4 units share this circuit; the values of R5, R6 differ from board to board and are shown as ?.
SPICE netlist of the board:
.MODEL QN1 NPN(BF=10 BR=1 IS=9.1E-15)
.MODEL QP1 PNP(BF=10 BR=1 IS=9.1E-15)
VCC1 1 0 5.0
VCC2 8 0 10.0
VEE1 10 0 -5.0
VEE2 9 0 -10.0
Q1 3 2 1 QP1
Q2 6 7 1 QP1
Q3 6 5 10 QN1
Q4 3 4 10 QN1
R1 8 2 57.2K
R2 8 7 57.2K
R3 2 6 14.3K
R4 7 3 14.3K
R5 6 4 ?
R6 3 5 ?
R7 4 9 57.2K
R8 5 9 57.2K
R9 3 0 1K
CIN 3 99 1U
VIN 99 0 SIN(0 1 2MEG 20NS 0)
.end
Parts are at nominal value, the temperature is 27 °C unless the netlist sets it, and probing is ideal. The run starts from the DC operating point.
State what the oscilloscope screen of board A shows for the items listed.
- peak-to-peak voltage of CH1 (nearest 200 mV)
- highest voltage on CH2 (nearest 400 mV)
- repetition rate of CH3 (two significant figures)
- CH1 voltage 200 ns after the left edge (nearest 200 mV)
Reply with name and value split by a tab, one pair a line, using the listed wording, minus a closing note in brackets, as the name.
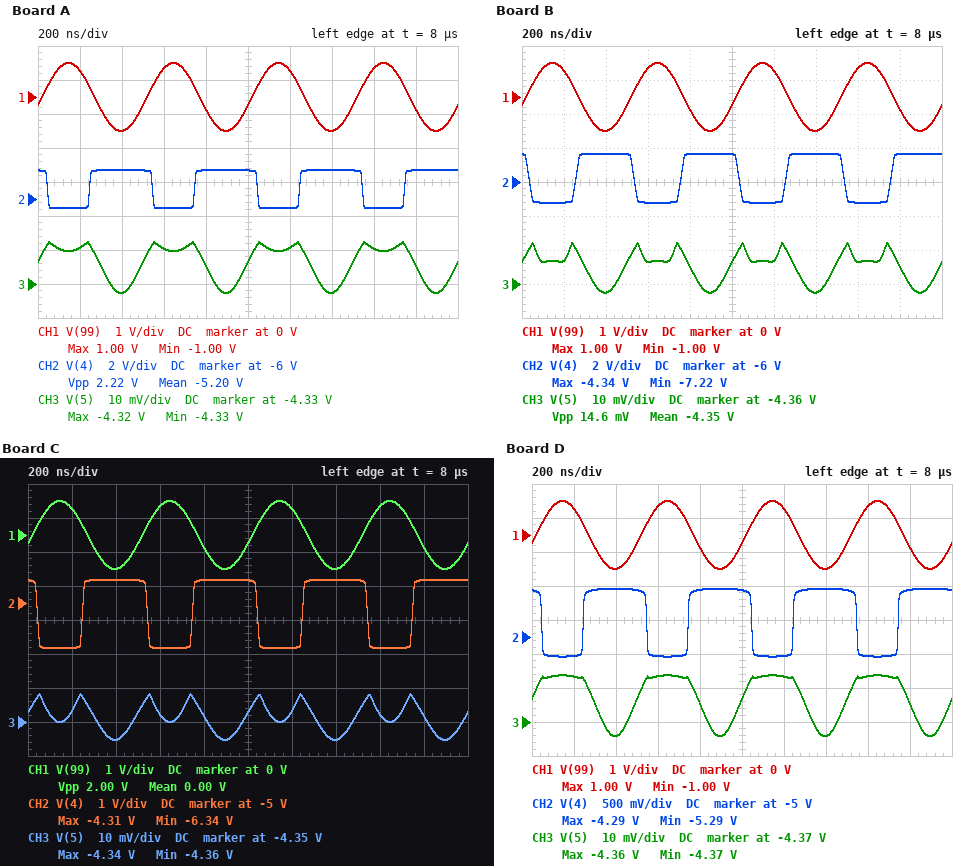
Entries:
peak-to-peak voltage of CH1	2.0 V
highest voltage on CH2	-4.4 V
repetition rate of CH3	2.0 MHz
CH1 voltage 200 ns after the left edge	800 mV
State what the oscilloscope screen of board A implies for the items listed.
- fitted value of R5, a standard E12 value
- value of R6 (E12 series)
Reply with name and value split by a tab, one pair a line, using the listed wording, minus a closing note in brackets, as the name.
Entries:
fitted value of R5, a standard E12 value	27 kΩ
value of R6	12 kΩ
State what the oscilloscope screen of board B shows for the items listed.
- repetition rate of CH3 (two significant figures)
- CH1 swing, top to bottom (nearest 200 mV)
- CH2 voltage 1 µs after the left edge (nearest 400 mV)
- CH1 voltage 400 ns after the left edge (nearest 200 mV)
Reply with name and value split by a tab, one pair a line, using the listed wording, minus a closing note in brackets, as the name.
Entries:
repetition rate of CH3	2.0 MHz
CH1 swing, top to bottom	2.0 V
CH2 voltage 1 µs after the left edge	-4.4 V
CH1 voltage 400 ns after the left edge	-1.0 V
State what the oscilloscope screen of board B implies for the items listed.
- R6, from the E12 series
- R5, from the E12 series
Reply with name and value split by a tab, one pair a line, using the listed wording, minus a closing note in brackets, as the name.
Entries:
R6, from the E12 series	39 kΩ
R5, from the E12 series	47 kΩ
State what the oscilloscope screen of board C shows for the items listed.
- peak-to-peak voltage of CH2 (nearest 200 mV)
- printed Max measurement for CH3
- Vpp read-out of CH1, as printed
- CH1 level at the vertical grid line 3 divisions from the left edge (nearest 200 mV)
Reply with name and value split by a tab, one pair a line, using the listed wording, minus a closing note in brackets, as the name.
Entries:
peak-to-peak voltage of CH2	2.0 V
printed Max measurement for CH3	-4.34 V
Vpp read-out of CH1, as printed	2.00 V
CH1 level at the vertical grid line 3 divisions from the left edge	800 mV
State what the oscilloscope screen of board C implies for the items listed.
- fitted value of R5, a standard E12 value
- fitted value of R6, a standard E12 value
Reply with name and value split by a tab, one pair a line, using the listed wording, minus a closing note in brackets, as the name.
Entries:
fitted value of R5, a standard E12 value	22 kΩ
fitted value of R6, a standard E12 value	33 kΩ
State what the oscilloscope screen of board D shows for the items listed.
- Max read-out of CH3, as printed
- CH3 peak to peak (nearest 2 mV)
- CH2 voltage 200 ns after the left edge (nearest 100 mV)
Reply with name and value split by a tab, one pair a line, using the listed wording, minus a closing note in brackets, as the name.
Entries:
Max read-out of CH3, as printed	-4.36 V
CH3 peak to peak	18 mV
CH2 voltage 200 ns after the left edge	-5.3 V
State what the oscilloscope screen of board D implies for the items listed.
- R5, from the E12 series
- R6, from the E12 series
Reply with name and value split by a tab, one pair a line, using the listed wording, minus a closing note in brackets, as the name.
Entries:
R5, from the E12 series	4.7 kΩ
R6, from the E12 series	47 kΩ
